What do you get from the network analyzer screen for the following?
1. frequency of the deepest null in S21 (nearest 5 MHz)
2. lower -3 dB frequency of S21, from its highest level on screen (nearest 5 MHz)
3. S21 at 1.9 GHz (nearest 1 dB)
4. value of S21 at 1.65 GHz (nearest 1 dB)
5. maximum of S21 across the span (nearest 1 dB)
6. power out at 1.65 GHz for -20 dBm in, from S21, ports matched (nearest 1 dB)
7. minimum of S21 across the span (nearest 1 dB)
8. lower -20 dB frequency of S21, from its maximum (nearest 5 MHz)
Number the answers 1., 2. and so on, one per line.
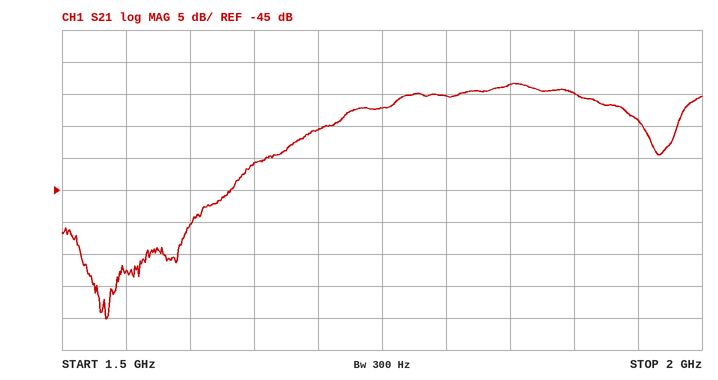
1. 1.535 GHz
2. 1.760 GHz
3. -30 dB
4. -41 dB
5. -28 dB
6. -61 dBm
7. -65 dB
8. 1.610 GHz
